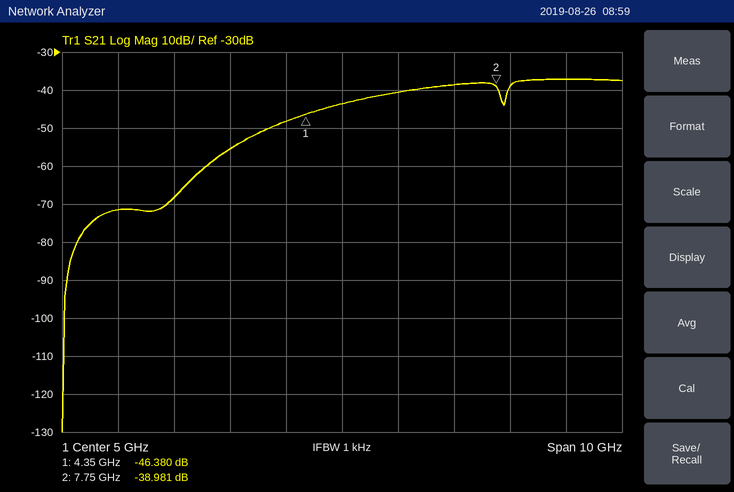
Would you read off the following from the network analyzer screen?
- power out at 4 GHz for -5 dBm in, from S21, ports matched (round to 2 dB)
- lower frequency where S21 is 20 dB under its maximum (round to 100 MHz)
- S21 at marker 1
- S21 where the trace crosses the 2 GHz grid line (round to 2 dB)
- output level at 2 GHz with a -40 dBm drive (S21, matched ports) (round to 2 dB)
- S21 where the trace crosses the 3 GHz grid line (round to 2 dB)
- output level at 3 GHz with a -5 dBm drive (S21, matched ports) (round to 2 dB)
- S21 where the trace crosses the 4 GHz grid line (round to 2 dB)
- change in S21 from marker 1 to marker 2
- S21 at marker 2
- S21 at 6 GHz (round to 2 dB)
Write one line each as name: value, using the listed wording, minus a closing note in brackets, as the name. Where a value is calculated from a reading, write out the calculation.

power out at 4 GHz for -5 dBm in, from S21, ports matched: -5 dBm + (-48 dB) = -54 dBm
lower frequency where S21 is 20 dB under its maximum: 2.8 GHz
S21 at marker 1: -46.380 dB
S21 where the trace crosses the 2 GHz grid line: -68 dB
output level at 2 GHz with a -40 dBm drive (S21, matched ports): -40 dBm + (-68 dB) = -108 dBm
S21 where the trace crosses the 3 GHz grid line: -56 dB
output level at 3 GHz with a -5 dBm drive (S21, matched ports): -5 dBm + (-56 dB) = -60 dBm
S21 where the trace crosses the 4 GHz grid line: -48 dB
change in S21 from marker 1 to marker 2: -38.981 − (-46.38) = 7.399 dB
S21 at marker 2: -38.981 dB
S21 at 6 GHz: -40 dB
